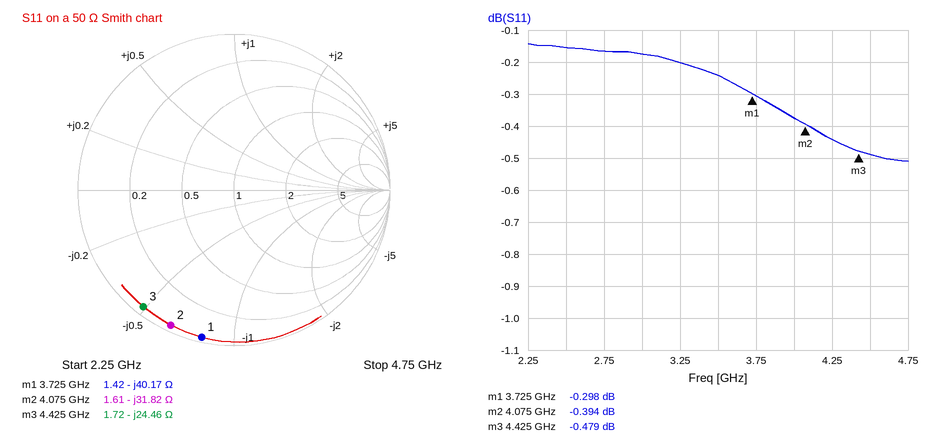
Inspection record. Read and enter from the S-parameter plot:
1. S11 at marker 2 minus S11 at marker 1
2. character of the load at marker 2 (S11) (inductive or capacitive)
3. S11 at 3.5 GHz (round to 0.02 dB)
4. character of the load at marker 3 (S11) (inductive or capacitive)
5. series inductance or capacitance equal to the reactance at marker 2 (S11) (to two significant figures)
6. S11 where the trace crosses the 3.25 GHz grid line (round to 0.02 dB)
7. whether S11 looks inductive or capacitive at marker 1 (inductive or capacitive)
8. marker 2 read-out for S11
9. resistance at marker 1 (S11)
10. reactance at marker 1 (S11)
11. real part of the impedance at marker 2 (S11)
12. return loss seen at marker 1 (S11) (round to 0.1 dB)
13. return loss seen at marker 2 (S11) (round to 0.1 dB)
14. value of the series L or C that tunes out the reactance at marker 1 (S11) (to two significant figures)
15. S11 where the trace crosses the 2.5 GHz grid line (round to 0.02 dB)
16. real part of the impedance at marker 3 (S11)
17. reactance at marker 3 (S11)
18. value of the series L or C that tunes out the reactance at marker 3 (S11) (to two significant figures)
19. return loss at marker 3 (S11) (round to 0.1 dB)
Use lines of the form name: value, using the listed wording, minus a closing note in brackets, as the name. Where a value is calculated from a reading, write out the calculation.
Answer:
S11 at marker 2 minus S11 at marker 1: -0.394 − (-0.298) = -0.096 dB
character of the load at marker 2 (S11): capacitive
S11 at 3.5 GHz: -0.24 dB
character of the load at marker 3 (S11): capacitive
series inductance or capacitance equal to the reactance at marker 2 (S11): C = 1/(2π × 4.075 GHz × 31.82 Ω) ≈ 1.2 pF
S11 where the trace crosses the 3.25 GHz grid line: -0.20 dB
whether S11 looks inductive or capacitive at marker 1: capacitive
marker 2 read-out for S11: -0.394 dB
resistance at marker 1: 1.42 Ω
reactance at marker 1: -40.17 Ω
real part of the impedance at marker 2: 1.61 Ω
return loss seen at marker 1 (S11): 0.3 dB
return loss seen at marker 2 (S11): 0.4 dB
value of the series L or C that tunes out the reactance at marker 1 (S11): L = 40.17 Ω/(2π × 3.725 GHz) ≈ 1.7 nH
S11 where the trace crosses the 2.5 GHz grid line: -0.16 dB
real part of the impedance at marker 3: 1.72 Ω
reactance at marker 3: -24.46 Ω
value of the series L or C that tunes out the reactance at marker 3 (S11): L = 24.46 Ω/(2π × 4.425 GHz) ≈ 880 pH
return loss at marker 3 (S11): 0.5 dB
